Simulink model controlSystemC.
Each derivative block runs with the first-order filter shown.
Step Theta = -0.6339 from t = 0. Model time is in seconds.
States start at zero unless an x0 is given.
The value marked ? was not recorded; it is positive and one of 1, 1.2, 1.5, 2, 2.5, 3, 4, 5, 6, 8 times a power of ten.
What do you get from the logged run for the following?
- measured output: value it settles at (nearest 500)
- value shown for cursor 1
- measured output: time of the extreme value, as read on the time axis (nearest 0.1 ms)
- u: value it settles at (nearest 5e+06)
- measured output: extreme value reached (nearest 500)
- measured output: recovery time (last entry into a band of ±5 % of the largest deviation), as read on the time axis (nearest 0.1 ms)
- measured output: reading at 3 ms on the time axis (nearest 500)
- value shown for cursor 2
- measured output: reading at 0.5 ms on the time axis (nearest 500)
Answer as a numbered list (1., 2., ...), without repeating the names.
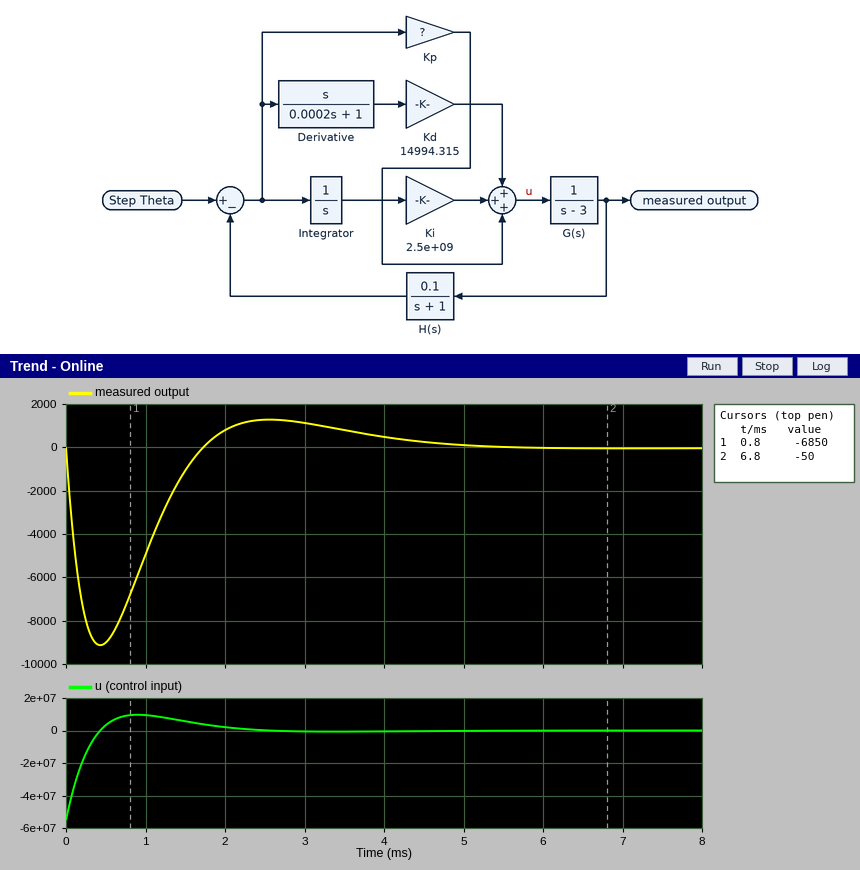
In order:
1. 0
2. -6850
3. 0.4 ms
4. 0
5. -9000
6. 4.1 ms
7. 1000
8. -50
9. -9000
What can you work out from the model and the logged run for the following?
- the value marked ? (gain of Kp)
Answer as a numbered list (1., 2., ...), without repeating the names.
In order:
1. 1.2e+07
